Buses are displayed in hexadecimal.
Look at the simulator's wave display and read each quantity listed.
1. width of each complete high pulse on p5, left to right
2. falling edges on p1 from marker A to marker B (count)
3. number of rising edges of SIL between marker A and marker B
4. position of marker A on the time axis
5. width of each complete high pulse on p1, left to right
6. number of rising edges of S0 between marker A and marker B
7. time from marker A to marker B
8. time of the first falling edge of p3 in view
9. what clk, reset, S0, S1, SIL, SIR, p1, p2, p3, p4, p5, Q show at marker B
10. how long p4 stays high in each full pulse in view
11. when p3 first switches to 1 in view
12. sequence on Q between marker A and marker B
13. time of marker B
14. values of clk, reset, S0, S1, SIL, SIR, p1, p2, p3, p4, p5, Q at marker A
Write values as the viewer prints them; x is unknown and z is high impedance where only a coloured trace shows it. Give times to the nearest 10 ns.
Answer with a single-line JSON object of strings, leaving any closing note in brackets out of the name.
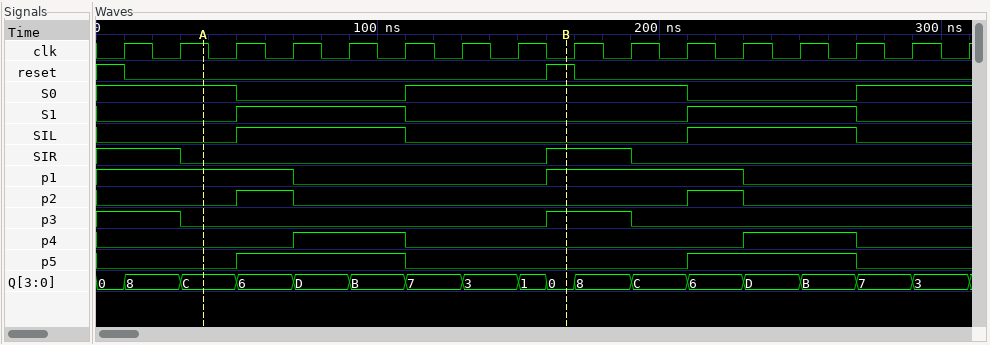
{"width of each complete high pulse on p5, left to right": "60 ns, 60 ns", "falling edges on p1 from marker A to marker B": "1", "number of rising edges of SIL between marker A and marker B": "1", "position of marker A on the time axis": "40 ns", "width of each complete high pulse on p1, left to right": "70 ns", "number of rising edges of S0 between marker A and marker B": "1", "time from marker A to marker B": "130 ns", "time of the first falling edge of p3 in view": "30 ns", "what clk, reset, S0, S1, SIL, SIR, p1, p2, p3, p4, p5, Q show at marker B": "clk=0, reset=1, S0=1, S1=0, SIL=0, SIR=1, p1=1, p2=0, p3=1, p4=0, p5=0, Q=0", "how long p4 stays high in each full pulse in view": "40 ns, 40 ns", "when p3 first switches to 1 in view": "160 ns", "sequence on Q between marker A and marker B": "C, 6, D, B, 7, 3, 1, 0", "time of marker B": "170 ns", "values of clk, reset, S0, S1, SIL, SIR, p1, p2, p3, p4, p5, Q at marker A": "clk=1, reset=0, S0=1, S1=0, SIL=0, SIR=0, p1=1, p2=0, p3=0, p4=0, p5=0, Q=C"}
